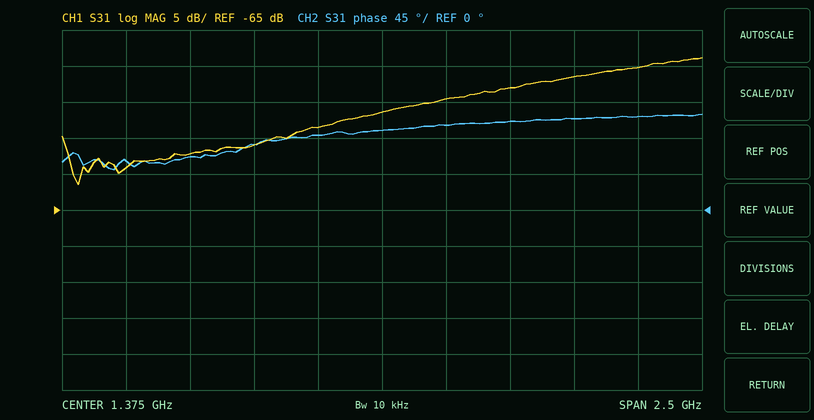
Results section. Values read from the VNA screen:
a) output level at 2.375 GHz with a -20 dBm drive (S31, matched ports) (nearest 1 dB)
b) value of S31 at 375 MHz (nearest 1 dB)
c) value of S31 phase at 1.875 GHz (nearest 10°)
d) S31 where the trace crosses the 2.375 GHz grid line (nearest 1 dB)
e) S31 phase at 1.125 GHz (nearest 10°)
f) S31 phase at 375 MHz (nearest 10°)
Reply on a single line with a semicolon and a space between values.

-65 dBm; -59 dB; 110°; -45 dB; 90°; 60°
